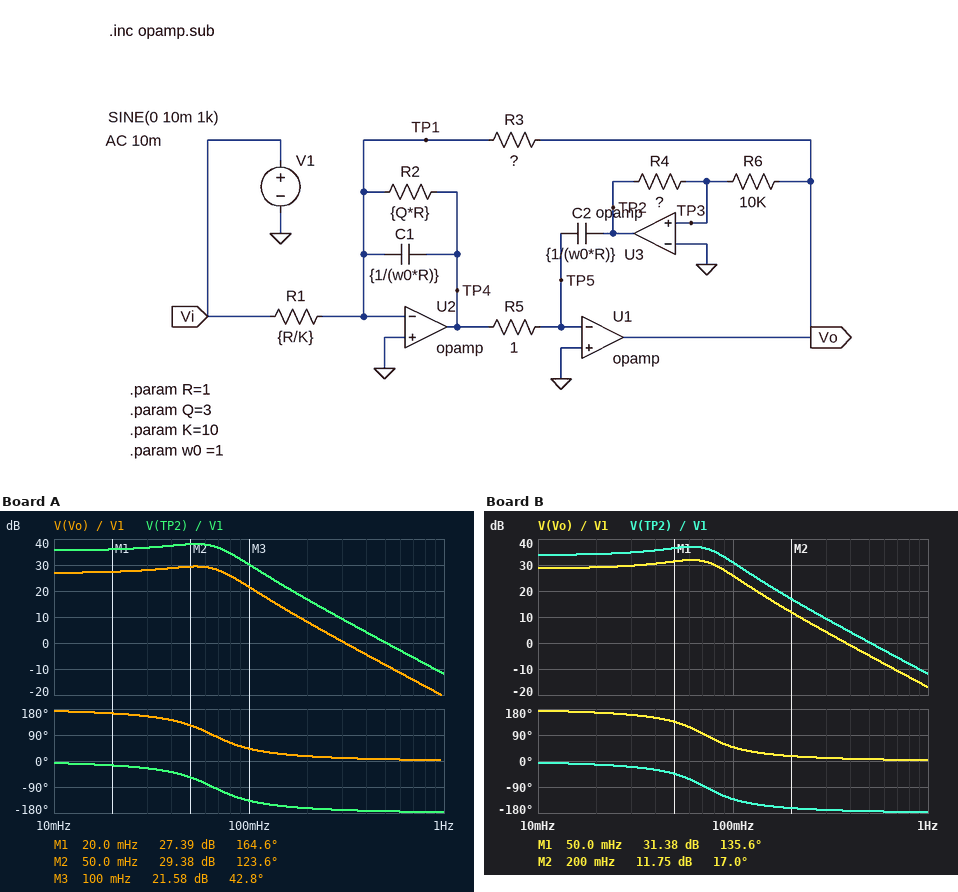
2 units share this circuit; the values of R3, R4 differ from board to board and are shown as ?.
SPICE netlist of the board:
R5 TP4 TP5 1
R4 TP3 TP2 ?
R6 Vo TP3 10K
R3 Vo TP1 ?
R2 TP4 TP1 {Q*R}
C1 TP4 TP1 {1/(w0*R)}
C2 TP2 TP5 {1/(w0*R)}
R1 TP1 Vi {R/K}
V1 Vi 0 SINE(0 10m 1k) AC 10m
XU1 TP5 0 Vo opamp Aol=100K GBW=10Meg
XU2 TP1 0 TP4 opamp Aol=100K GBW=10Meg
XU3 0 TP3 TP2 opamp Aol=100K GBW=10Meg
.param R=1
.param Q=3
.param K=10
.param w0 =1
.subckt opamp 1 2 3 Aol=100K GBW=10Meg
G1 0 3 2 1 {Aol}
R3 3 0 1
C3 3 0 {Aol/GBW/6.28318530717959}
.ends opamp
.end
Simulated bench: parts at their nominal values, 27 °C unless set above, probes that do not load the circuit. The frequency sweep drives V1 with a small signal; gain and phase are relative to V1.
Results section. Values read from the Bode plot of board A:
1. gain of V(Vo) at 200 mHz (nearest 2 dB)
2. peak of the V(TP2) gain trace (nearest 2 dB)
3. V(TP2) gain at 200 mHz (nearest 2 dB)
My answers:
8 dB
38 dB
16 dB
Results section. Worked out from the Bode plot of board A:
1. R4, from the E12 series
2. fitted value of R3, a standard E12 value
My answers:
27 kΩ
2.2 Ω
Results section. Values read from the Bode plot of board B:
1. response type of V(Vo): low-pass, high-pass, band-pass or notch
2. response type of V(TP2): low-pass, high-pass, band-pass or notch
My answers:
low-pass
low-pass
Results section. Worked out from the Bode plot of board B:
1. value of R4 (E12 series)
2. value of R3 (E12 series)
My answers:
18 kΩ
2.7 Ω
